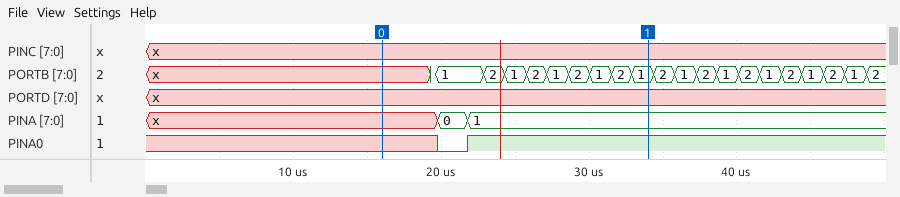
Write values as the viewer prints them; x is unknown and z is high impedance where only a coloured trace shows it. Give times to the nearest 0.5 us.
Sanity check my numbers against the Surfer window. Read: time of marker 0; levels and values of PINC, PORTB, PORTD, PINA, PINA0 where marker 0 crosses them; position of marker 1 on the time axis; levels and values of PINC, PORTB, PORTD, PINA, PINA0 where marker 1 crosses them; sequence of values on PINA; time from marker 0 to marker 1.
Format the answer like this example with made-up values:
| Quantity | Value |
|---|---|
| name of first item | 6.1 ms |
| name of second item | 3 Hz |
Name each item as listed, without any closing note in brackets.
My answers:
| Quantity | Value |
|---|---|
| time of marker 0 | 16 us |
| levels and values of PINC, PORTB, PORTD, PINA, PINA0 where marker 0 crosses them | PINC=x, PORTB=x, PORTD=x, PINA=x, PINA0=x |
| position of marker 1 on the time axis | 34 us |
| levels and values of PINC, PORTB, PORTD, PINA, PINA0 where marker 1 crosses them | PINC=x, PORTB=1, PORTD=x, PINA=1, PINA0=1 |
| sequence of values on PINA | x, 0, 1 |
| time from marker 0 to marker 1 | 18 us |
